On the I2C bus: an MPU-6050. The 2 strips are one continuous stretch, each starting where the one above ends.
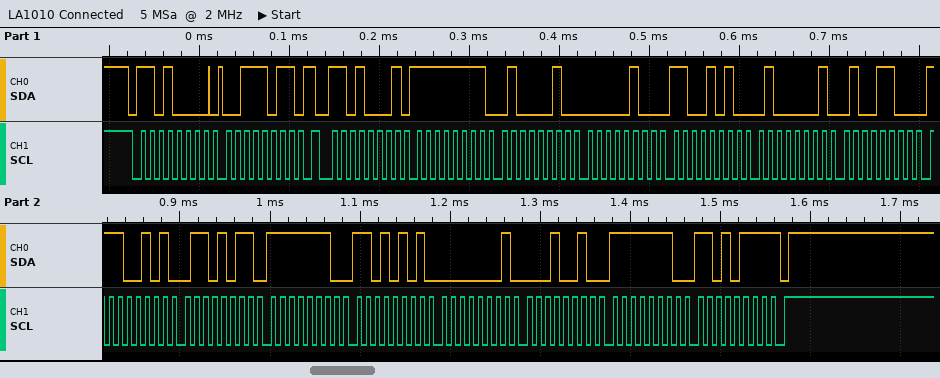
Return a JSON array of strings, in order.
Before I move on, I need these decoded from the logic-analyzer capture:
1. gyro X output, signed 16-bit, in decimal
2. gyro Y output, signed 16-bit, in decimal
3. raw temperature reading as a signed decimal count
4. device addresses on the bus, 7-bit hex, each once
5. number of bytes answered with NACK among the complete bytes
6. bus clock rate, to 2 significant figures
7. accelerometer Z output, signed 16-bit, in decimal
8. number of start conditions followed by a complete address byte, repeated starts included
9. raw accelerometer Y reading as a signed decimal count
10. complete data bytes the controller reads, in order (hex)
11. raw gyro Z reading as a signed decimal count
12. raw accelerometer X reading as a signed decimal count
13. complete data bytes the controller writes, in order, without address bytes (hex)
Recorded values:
["-299", "274", "-6805", "0x68", "1", "100 kHz", "16716", "2", "1226", "FF 42 04 CA 41 4C E5 6B FE D5 01 12 FE D7", "-297", "-190", "3B"]
